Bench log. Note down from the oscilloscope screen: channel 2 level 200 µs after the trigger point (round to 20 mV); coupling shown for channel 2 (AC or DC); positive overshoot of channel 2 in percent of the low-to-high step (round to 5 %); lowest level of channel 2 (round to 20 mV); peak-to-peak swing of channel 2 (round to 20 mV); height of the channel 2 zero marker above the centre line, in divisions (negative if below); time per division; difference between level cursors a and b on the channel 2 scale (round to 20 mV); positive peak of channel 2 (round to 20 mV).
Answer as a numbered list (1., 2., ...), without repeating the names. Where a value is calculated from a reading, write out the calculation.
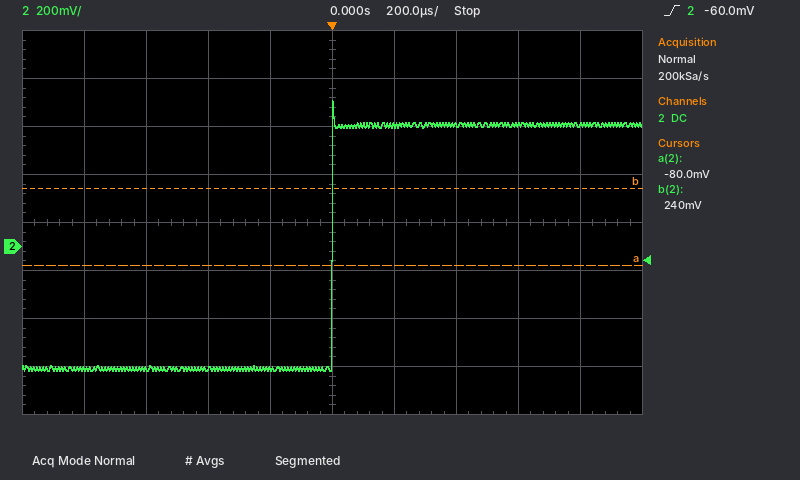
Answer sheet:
1. 500 mV
2. DC
3. 10 %
4. -520 mV
5. 600 mV − (-520 mV) = 1.12 V
6. -0.5 div
7. 200 µs
8. 320 mV
9. 600 mV
